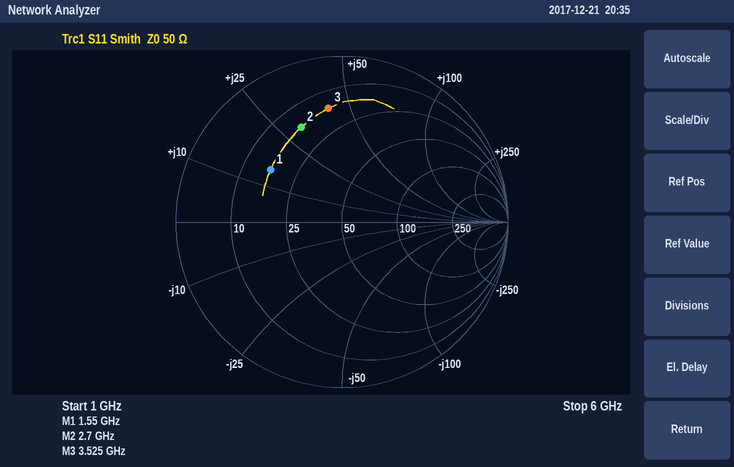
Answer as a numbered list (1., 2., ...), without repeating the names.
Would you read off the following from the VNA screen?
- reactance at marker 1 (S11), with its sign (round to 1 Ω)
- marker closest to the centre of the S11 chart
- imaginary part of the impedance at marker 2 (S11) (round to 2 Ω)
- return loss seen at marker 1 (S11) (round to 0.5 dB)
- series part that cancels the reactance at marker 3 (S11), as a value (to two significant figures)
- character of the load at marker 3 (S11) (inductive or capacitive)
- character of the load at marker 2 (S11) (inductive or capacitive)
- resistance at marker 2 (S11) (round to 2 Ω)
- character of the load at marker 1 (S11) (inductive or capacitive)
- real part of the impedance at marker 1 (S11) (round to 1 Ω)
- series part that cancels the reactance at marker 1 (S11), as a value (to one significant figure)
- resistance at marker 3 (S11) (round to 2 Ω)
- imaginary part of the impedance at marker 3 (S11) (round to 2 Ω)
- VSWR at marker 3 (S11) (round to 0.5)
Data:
1. +15 Ω
2. marker 1
3. +30 Ω
4. 5.5 dB
5. 1.1 pF
6. inductive
7. inductive
8. 16 Ω
9. inductive
10. 17 Ω
11. 7 pF
12. 16 Ω
13. +42 Ω
14. 5.5
